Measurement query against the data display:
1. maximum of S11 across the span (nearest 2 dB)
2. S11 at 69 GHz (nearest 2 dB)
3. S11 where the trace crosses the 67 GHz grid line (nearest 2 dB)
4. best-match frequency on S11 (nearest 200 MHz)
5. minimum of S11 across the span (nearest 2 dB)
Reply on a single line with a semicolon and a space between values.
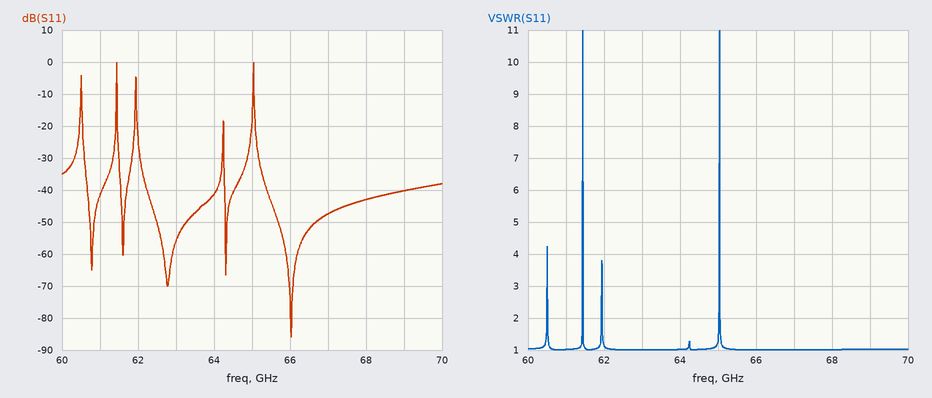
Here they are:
0 dB; -40 dB; -48 dB; 66.0 GHz; -86 dB
